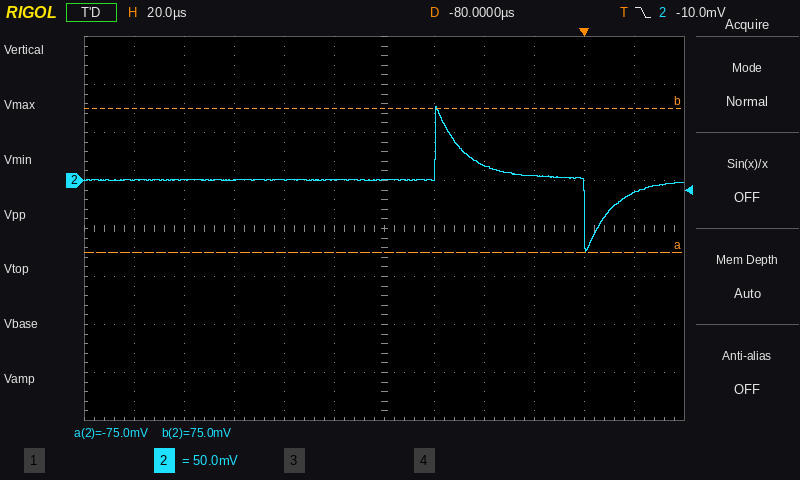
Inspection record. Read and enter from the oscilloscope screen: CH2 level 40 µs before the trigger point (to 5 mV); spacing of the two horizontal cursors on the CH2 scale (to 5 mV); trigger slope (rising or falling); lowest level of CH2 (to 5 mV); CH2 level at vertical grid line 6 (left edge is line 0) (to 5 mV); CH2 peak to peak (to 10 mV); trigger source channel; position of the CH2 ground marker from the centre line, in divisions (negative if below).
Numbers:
15 mV
150 mV
falling
-75 mV
0 mV
150 mV
CH2
+1.0 div
